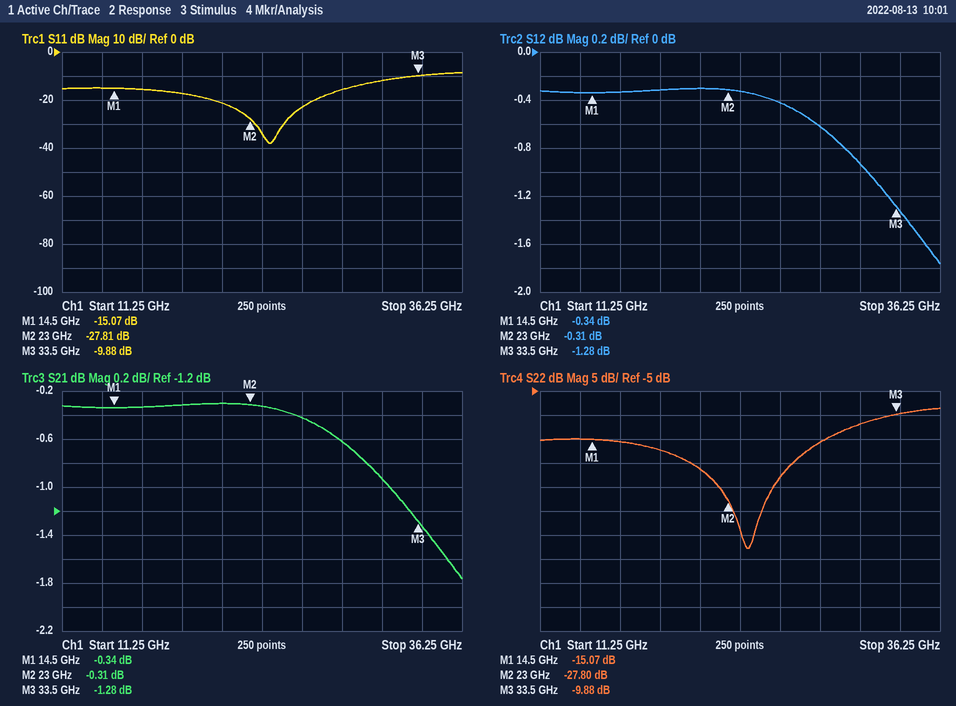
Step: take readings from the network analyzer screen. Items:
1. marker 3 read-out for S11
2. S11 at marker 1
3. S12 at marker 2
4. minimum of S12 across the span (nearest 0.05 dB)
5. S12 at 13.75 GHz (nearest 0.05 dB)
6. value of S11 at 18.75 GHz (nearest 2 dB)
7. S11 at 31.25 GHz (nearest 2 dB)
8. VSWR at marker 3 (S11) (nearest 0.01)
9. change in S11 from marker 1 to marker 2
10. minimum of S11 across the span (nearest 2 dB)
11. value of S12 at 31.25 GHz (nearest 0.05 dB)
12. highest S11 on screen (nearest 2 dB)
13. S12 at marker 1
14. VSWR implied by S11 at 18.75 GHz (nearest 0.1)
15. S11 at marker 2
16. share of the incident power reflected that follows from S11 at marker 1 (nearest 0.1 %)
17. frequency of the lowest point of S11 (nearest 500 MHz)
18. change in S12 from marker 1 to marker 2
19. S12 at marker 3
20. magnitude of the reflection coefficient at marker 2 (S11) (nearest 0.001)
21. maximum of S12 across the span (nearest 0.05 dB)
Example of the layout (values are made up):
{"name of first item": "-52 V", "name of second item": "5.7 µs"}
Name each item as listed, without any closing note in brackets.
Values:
{"marker 3 read-out for S11": "-9.88 dB", "S11 at marker 1": "-15.07 dB", "S12 at marker 2": "-0.31 dB", "minimum of S12 across the span": "-1.75 dB", "S12 at 13.75 GHz": "-0.35 dB", "value of S11 at 18.75 GHz": "-18 dB", "S11 at 31.25 GHz": "-12 dB", "VSWR at marker 3 (S11)": "1.94", "change in S11 from marker 1 to marker 2": "-12.74 dB", "minimum of S11 across the span": "-38 dB", "value of S12 at 31.25 GHz": "-0.95 dB", "highest S11 on screen": "-8 dB", "S12 at marker 1": "-0.34 dB", "VSWR implied by S11 at 18.75 GHz": "1.3", "S11 at marker 2": "-27.81 dB", "share of the incident power reflected that follows from S11 at marker 1": "3.1 %", "frequency of the lowest point of S11": "24.0 GHz", "change in S12 from marker 1 to marker 2": "0.03 dB", "S12 at marker 3": "-1.28 dB", "magnitude of the reflection coefficient at marker 2 (S11)": "0.041", "maximum of S12 across the span": "-0.30 dB"}
